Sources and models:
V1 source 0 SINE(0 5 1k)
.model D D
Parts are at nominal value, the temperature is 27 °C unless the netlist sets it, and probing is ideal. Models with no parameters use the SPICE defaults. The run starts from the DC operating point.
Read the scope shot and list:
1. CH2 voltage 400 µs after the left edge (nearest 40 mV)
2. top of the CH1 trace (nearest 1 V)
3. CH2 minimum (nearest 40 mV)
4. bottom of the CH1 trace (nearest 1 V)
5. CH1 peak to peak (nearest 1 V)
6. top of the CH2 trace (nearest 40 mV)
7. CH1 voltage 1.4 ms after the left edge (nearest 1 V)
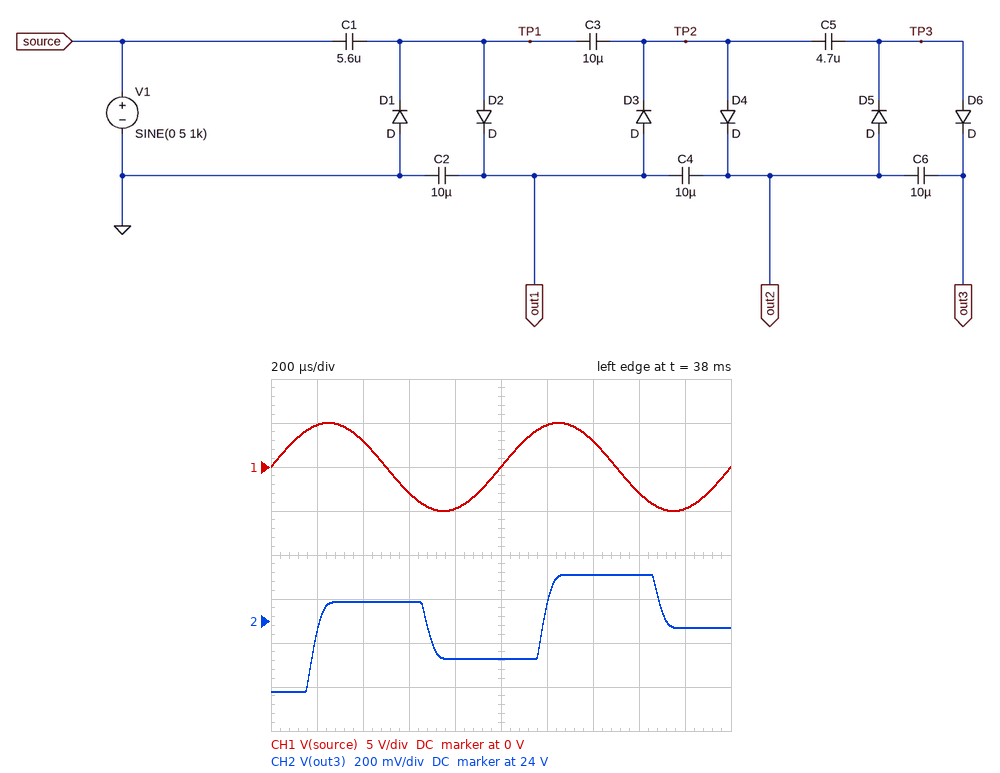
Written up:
24.08 V
5 V
23.68 V
-5 V
10 V
24.20 V
3 V
